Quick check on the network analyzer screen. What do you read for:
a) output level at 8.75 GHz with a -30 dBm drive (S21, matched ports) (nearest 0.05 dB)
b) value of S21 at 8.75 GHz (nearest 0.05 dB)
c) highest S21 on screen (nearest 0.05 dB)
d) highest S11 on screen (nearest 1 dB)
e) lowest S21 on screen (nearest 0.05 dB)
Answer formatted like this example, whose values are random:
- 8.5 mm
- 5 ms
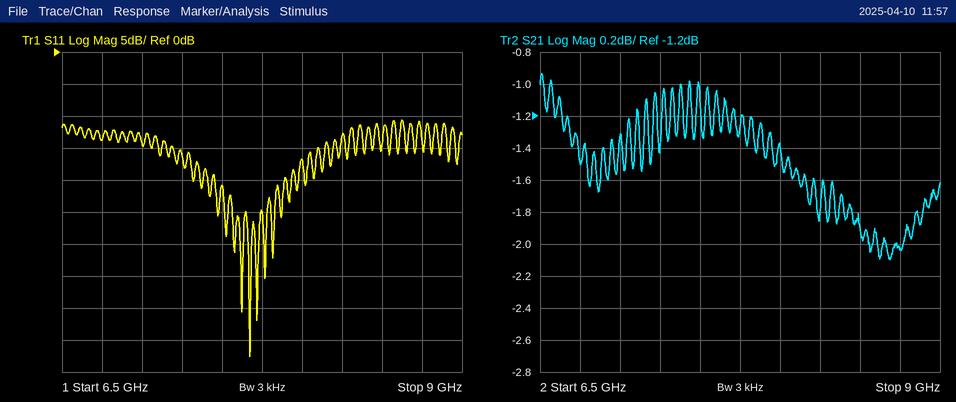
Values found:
- -32.05 dBm
- -2.05 dB
- -0.95 dB
- -11 dB
- -2.10 dB
